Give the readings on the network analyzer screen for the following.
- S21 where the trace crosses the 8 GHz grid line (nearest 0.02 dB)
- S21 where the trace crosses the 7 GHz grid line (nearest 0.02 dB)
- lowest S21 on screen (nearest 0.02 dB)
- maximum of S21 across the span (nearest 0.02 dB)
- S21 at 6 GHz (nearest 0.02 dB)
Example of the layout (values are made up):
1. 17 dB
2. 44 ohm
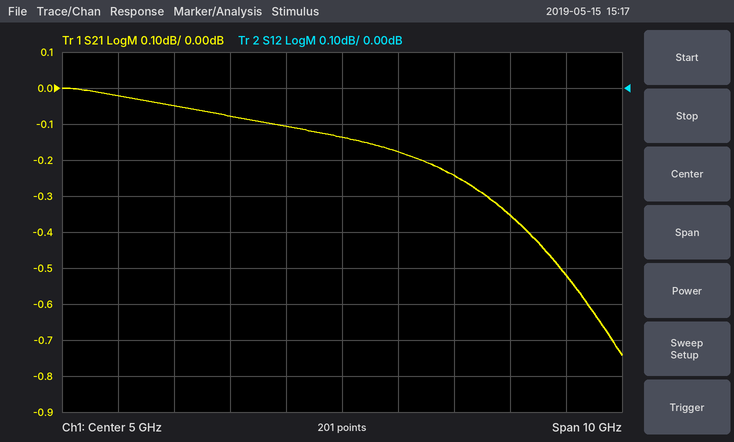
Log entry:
1. -0.36 dB
2. -0.24 dB
3. -0.74 dB
4. 0.00 dB
5. -0.18 dB
